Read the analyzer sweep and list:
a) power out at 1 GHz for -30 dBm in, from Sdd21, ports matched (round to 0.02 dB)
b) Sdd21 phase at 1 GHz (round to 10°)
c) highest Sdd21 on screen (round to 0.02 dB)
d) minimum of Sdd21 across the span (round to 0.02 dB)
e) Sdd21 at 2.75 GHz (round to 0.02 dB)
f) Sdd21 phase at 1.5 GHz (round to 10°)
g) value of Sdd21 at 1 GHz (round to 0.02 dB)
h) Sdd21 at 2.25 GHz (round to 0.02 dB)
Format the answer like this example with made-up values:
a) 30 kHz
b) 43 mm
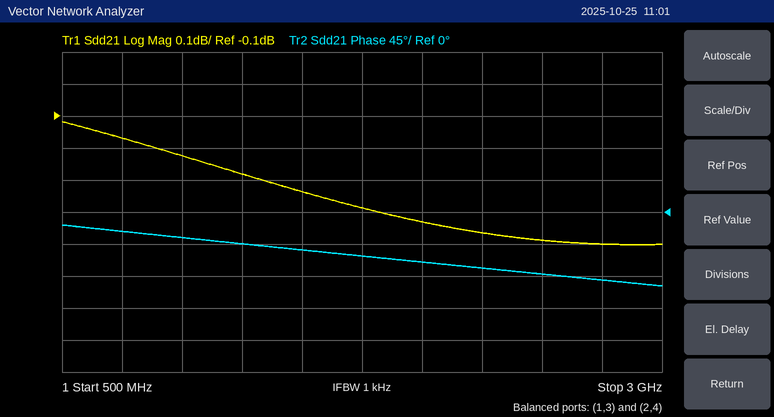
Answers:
a) -30.22 dBm
b) -40°
c) -0.12 dB
d) -0.50 dB
e) -0.50 dB
f) -50°
g) -0.22 dB
h) -0.46 dB
